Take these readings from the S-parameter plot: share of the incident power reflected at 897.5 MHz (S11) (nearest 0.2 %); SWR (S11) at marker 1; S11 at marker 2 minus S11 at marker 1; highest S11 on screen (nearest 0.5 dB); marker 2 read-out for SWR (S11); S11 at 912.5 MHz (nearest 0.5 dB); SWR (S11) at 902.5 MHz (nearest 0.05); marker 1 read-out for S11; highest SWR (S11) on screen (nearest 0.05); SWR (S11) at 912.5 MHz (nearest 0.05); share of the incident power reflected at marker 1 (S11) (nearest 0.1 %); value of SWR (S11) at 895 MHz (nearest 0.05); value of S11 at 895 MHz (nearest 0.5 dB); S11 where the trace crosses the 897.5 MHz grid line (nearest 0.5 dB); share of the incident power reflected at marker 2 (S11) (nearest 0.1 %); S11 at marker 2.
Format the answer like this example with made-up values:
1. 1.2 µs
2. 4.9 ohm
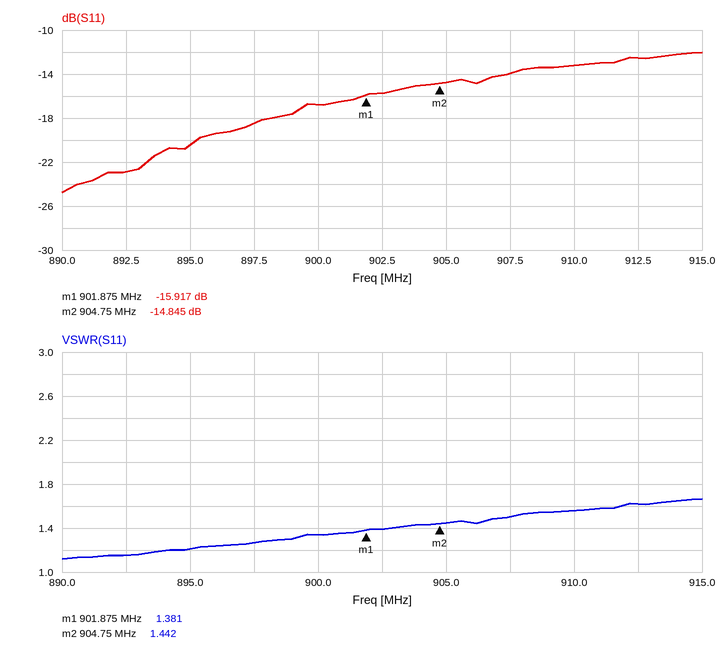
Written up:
1. 1.4 %
2. 1.381
3. 1.072 dB
4. -12.0 dB
5. 1.442
6. -12.5 dB
7. 1.40
8. -15.917 dB
9. 1.65
10. 1.60
11. 2.6 %
12. 1.20
13. -20.5 dB
14. -18.5 dB
15. 3.3 %
16. -14.845 dB
